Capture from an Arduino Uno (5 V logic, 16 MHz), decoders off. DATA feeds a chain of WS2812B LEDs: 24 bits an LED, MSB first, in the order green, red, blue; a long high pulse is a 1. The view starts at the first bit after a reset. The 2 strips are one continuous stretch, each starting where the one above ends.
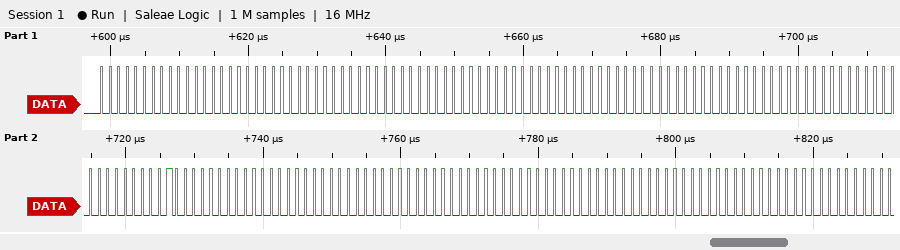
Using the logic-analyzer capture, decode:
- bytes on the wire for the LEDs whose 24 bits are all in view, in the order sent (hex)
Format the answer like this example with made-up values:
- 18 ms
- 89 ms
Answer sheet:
- 00 00 00 00 00 00 00 00 00 00 00 00 02 00 00 00 00 00 00 00 00
